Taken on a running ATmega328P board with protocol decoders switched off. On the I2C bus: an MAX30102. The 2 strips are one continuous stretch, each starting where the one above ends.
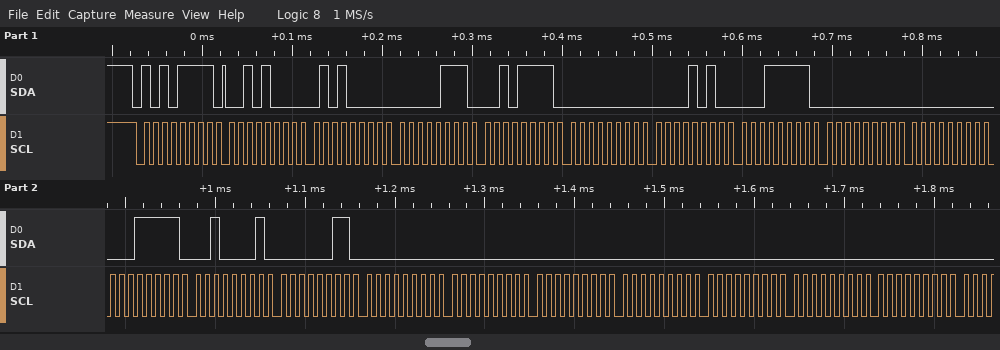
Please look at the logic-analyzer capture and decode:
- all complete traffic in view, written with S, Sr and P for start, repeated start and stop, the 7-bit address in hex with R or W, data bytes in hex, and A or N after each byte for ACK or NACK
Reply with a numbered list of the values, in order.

1. S 57R A 28 A 50 A 07 A 2F A 00 A 0A A 1F A 00 A 00 A 1F A 21 A 03 A 00 A 00 A 00 A 00 A 00 A 00 A 00 A
